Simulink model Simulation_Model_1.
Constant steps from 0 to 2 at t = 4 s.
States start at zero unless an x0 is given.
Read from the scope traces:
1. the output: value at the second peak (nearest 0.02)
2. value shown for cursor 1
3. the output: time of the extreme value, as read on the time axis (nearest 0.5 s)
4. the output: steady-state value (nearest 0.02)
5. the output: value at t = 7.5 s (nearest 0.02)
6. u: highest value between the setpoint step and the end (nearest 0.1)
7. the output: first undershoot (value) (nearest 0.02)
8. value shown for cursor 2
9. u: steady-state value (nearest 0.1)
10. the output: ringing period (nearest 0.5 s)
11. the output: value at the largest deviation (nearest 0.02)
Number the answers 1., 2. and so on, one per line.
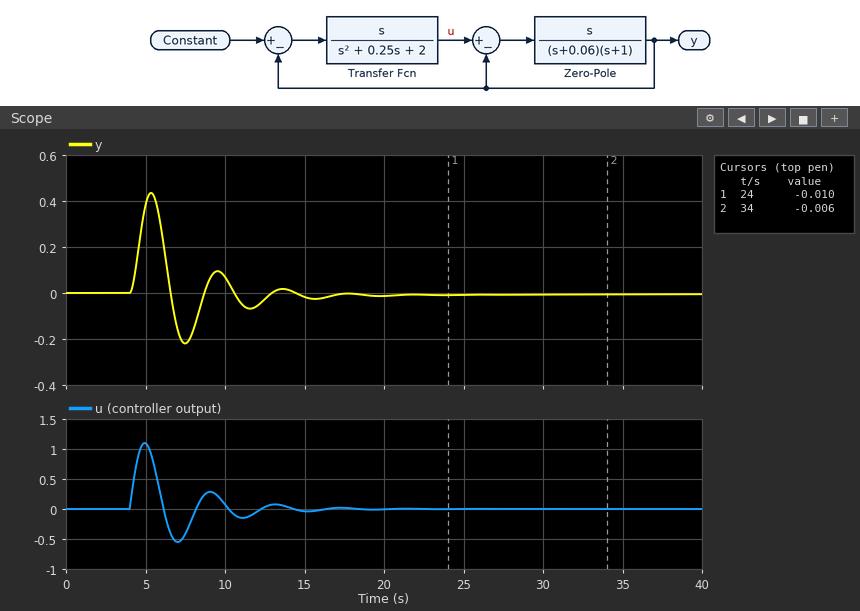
1. 0.10
2. -0.010
3. 5.5 s
4. 0.00
5. -0.22
6. 1.1
7. -0.22
8. -0.006
9. 0.0
10. 4.0 s
11. 0.44
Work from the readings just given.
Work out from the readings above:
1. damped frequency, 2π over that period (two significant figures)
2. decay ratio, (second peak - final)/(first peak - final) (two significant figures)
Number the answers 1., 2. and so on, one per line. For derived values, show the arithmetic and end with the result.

1. 2π / 4 = 1.6 rad/s
2. (0.1 - 0) / (0.44 - 0) = 0.23
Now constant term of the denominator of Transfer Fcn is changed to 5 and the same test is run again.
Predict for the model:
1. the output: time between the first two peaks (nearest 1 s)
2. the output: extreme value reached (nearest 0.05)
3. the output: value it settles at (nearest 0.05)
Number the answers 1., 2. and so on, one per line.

1. 3 s
2. 0.25
3. 0.00
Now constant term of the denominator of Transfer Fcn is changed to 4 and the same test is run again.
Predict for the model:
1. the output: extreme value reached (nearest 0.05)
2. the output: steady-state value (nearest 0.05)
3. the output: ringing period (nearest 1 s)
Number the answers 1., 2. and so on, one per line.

1. 0.30
2. 0.00
3. 3 s
